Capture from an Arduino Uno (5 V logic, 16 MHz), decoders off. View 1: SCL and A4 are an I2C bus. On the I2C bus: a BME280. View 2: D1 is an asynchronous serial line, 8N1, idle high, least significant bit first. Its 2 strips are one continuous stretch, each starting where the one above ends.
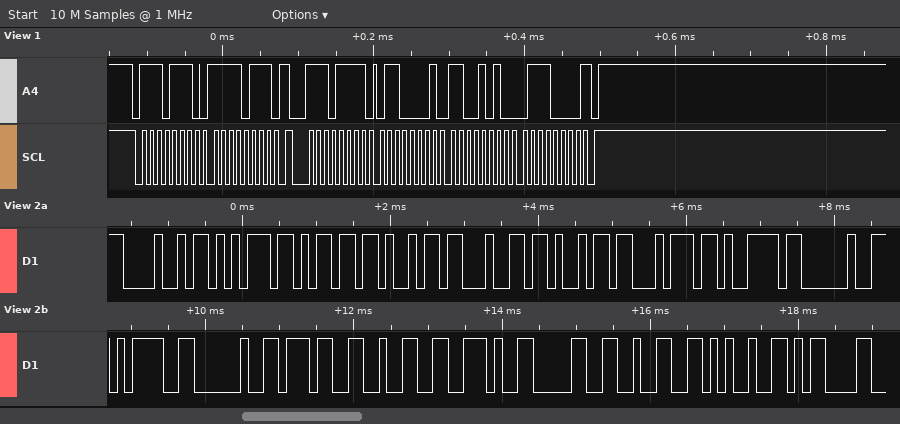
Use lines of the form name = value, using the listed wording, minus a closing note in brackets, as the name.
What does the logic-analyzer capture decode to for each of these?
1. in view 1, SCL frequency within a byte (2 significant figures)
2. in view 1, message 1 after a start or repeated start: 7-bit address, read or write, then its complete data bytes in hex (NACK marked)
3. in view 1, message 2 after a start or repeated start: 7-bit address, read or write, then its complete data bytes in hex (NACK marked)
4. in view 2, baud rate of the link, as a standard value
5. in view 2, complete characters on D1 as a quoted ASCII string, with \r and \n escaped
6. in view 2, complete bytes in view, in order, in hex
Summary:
in view 1, SCL frequency within a byte = 100 kHz
in view 1, message 1 after a start or repeated start: 7-bit address, read or write, then its complete data bytes in hex = 0x77 write: F7
in view 1, message 2 after a start or repeated start: 7-bit address, read or write, then its complete data bytes in hex = 0x77 read: 61 CA 70 NACK
in view 2, baud rate of the link, as a standard value = 9600 baud
in view 2, complete characters on D1 as a quoted ASCII string, with \r and \n escaped = "Humidity = 72.02%\r"
in view 2, complete bytes in view, in order, in hex = 48 75 6D 69 64 69 74 79 20 3D 20 37 32 2E 30 32 25 0D
